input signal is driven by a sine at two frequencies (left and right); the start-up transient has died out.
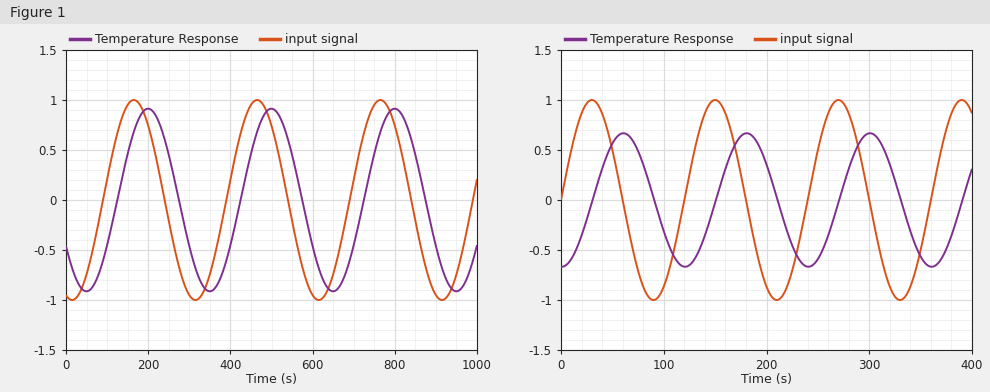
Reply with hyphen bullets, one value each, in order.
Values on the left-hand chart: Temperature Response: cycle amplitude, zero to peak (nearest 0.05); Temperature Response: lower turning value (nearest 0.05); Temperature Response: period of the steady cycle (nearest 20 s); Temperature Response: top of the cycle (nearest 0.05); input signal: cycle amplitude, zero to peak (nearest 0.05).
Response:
- 0.90
- -0.90
- 300 s
- 0.90
- 1.00
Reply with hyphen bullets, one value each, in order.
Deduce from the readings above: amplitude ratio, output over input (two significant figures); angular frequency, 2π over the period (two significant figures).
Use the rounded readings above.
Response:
- 0.90
- 0.021 rad/s
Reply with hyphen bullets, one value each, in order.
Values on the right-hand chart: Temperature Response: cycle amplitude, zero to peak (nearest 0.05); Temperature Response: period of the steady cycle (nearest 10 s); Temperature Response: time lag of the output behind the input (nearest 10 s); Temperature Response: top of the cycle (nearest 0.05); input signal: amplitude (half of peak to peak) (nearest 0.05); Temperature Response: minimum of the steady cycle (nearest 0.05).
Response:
- 0.65
- 120 s
- 30 s
- 0.65
- 1.00
- -0.65
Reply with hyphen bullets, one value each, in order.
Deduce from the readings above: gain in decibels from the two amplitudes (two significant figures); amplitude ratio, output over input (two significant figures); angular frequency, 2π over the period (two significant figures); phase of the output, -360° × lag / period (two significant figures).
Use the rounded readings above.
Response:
- -3.7 dB
- 0.65
- 0.052 rad/s
- -90°
